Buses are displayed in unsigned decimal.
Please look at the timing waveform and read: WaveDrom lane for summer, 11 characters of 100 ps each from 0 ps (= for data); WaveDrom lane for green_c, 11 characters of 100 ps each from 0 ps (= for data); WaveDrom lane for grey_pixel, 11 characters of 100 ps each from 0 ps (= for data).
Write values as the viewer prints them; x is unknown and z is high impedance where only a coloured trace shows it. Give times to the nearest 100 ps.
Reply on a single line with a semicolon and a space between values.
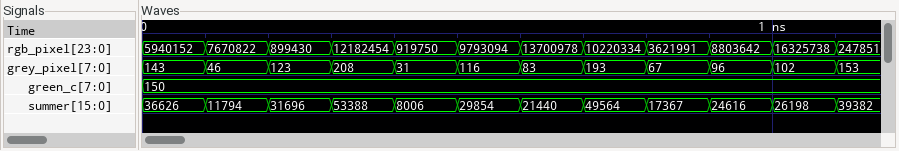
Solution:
{name: 'summer', wave: '===========', data: '36626 11794 31696 53388 8006 29854 21440 49564 17367 24616 26198'}; {name: 'green_c', wave: '=..........', data: '150'}; {name: 'grey_pixel', wave: '===========', data: '143 46 123 208 31 116 83 193 67 96 102'}
